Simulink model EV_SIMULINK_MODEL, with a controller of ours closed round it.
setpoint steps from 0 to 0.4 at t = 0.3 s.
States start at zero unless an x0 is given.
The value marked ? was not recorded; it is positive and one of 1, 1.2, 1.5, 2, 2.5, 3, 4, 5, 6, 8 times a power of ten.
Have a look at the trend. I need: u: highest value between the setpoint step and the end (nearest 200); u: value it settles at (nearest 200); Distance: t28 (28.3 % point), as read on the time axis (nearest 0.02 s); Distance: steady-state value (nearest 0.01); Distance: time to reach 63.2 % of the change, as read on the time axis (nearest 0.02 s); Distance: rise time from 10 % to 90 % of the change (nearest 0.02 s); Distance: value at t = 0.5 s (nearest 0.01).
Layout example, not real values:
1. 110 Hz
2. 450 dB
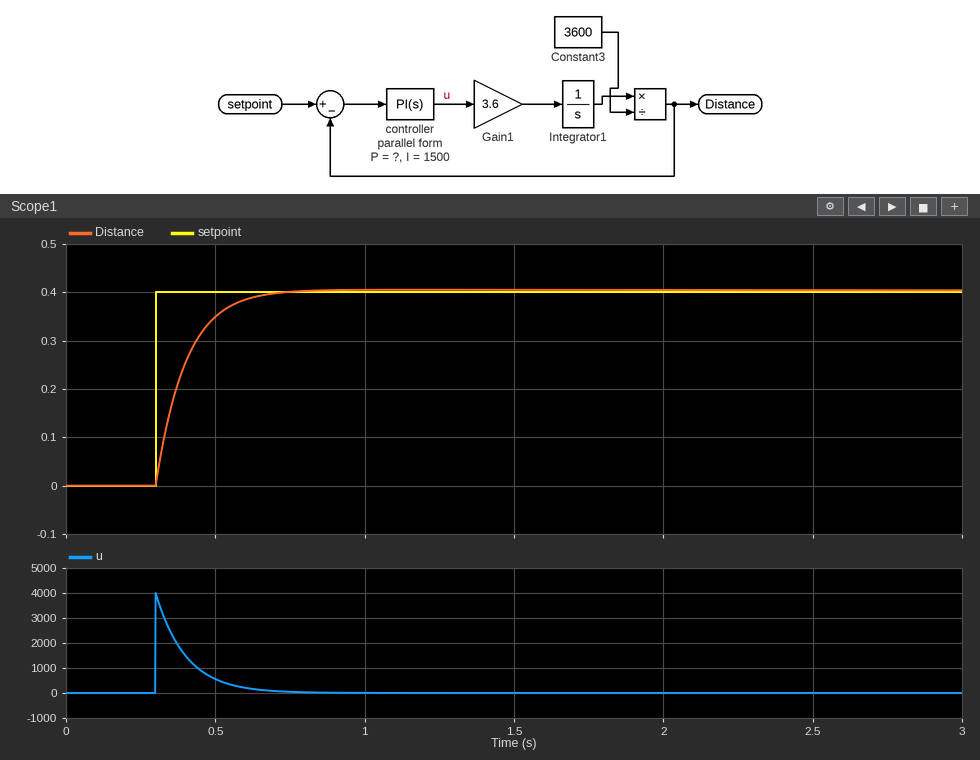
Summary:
1. 4000
2. 0
3. 0.34 s
4. 0.40
5. 0.40 s
6. 0.22 s
7. 0.35
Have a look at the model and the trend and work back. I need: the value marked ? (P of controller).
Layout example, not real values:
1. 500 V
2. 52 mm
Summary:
1. 10000
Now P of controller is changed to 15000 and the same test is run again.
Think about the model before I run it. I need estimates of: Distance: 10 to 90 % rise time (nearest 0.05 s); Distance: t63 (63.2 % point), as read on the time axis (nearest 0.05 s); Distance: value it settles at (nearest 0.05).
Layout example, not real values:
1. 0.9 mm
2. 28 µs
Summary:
1. 0.15 s
2. 0.35 s
3. 0.40
